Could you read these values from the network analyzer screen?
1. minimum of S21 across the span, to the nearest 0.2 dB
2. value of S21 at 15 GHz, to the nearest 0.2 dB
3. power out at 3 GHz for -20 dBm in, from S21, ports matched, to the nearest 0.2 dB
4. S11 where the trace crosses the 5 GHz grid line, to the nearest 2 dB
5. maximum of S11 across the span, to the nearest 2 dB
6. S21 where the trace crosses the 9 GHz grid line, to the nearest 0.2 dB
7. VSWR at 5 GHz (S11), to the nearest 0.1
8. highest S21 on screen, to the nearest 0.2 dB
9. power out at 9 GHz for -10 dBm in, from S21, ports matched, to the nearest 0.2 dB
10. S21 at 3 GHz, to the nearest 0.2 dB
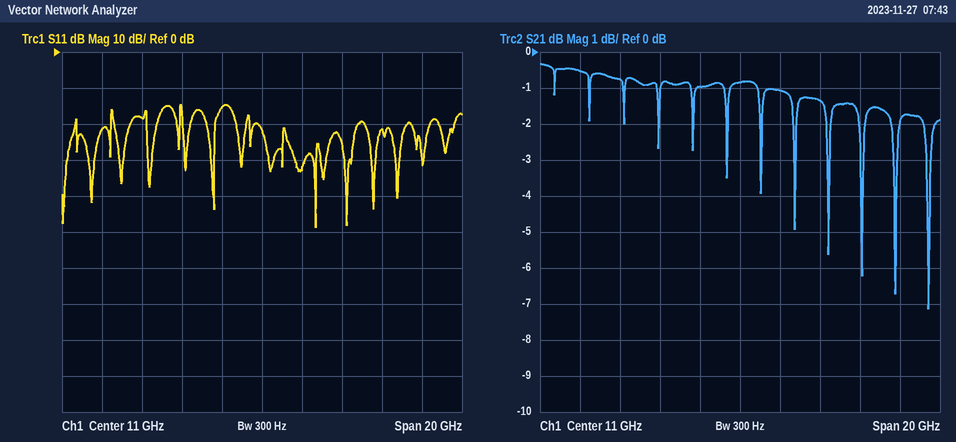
-7.2 dB
-1.4 dB
-20.6 dBm
-18 dB
-14 dB
-1.0 dB
1.3
-0.4 dB
-11.0 dBm
-0.6 dB
